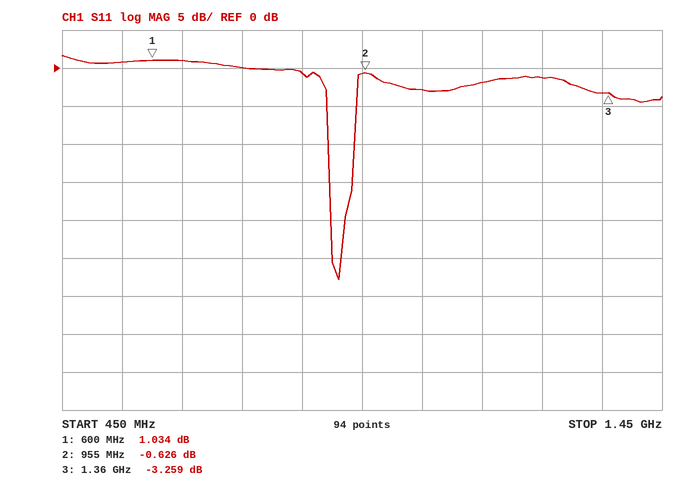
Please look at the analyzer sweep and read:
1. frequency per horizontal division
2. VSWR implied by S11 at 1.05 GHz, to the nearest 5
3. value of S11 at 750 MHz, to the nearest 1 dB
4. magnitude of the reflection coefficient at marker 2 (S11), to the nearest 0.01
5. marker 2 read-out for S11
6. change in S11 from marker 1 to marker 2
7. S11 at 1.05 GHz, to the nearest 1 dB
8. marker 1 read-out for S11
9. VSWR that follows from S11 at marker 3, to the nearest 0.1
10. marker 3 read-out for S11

100 MHz
5
0 dB
0.93
-0.626 dB
-1.660 dB
-3 dB
1.034 dB
5.4
-3.259 dB
